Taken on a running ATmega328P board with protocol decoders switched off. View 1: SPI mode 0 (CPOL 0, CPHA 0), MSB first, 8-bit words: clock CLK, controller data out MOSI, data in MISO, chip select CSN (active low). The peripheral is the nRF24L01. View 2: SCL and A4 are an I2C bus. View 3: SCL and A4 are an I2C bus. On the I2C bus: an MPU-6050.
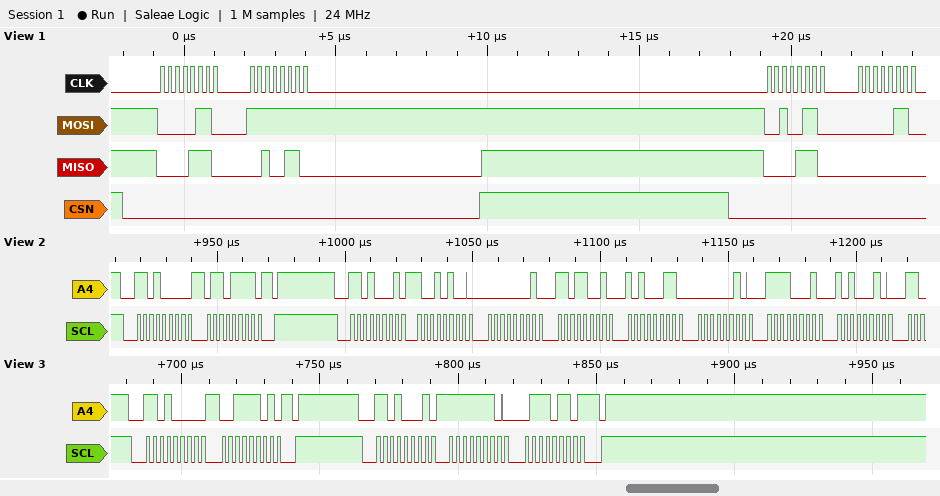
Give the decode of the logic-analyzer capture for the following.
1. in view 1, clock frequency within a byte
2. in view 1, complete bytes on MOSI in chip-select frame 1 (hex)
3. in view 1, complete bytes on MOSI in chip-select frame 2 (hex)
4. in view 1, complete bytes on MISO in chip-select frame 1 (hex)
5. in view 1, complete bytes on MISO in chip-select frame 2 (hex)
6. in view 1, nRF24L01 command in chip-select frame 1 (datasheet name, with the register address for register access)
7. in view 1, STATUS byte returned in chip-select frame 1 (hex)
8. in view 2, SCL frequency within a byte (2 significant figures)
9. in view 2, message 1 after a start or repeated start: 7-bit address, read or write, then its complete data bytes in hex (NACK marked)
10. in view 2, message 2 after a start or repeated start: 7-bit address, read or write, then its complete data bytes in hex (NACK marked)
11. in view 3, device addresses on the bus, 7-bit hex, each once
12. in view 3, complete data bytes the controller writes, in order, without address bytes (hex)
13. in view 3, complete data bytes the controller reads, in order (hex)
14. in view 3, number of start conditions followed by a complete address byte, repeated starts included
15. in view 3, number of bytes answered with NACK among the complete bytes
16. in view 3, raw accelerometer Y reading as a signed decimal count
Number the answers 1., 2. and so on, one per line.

1. 4 MHz
2. 06 FF
3. 26 06
4. 0E 26
5. 0E 00
6. R_REGISTER 0x06
7. 0x0E
8. 400 kHz
9. 0x68 write: 6F
10. 0x68 read: 94 01 D9 A3 02 F1 A2
11. 0x68
12. 3D
13. FE 76
14. 2
15. 1
16. -394
